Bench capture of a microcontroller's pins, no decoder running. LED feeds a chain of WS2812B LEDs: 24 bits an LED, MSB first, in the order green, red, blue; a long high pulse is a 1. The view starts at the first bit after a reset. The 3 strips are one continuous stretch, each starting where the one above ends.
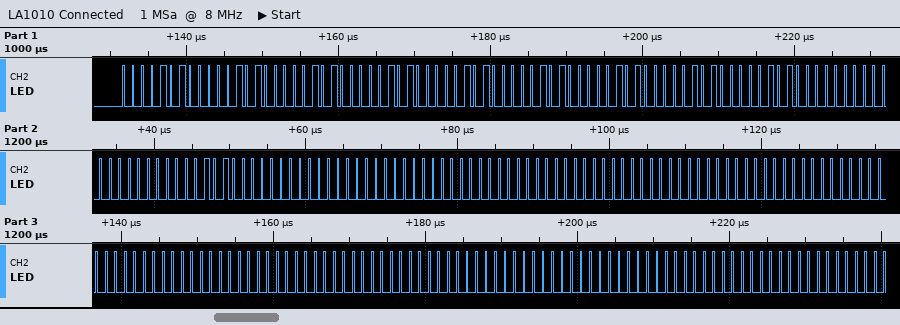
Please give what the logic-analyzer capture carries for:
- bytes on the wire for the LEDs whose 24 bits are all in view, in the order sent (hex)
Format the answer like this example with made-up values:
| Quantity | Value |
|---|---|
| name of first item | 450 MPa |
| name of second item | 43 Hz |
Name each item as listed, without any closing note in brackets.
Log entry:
| Quantity | Value |
|---|---|
| bytes on the wire for the LEDs whose 24 bits are all in view, in the order sent | 0A 0A 0A 0A 0A 0A 0A 0A 0A 00 00 0A 00 00 00 00 00 00 00 00 00 00 00 00 00 00 00 00 00 00 |
